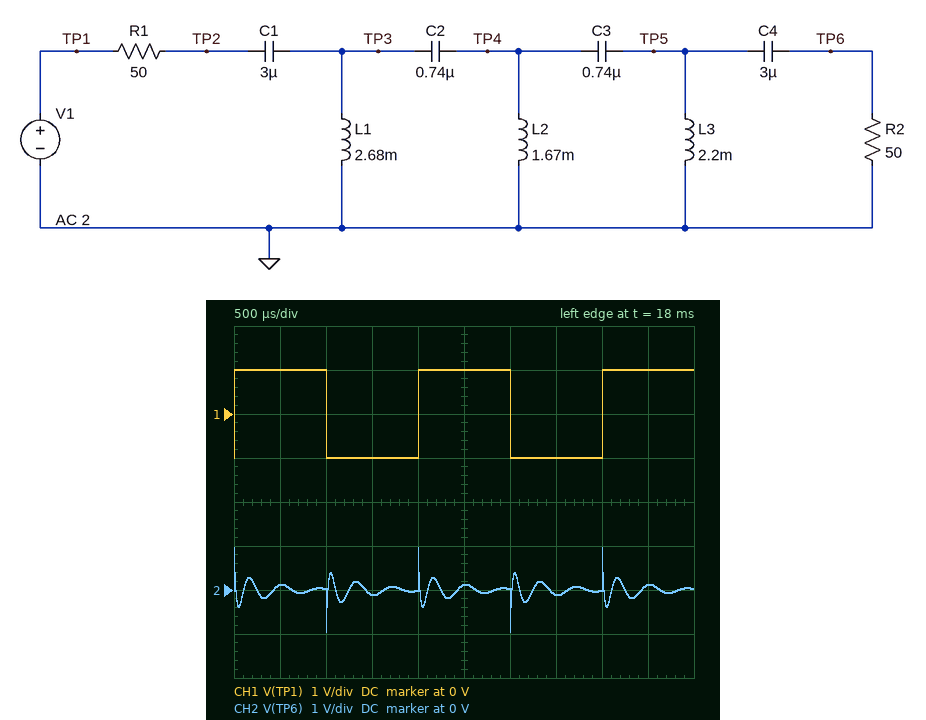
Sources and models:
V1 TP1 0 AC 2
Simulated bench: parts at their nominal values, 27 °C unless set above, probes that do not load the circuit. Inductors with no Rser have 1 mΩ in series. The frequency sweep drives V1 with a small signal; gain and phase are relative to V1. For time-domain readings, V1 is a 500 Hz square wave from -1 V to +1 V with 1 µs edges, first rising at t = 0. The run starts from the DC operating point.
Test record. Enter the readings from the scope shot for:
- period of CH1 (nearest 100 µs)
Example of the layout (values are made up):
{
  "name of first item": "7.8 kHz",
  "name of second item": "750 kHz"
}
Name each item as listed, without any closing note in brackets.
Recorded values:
{
  "period of CH1": "2.0 ms"
}
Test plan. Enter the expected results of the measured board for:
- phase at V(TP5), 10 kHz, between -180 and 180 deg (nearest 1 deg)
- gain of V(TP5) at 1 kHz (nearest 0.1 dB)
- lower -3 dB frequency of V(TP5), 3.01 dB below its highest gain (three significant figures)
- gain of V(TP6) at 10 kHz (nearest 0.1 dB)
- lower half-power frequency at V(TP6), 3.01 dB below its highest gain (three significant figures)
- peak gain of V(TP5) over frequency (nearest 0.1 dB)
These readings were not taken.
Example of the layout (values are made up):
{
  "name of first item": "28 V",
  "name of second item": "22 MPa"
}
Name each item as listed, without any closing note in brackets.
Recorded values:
{
  "phase at V(TP5), 10 kHz, between -180 and 180 deg": "58 deg",
  "gain of V(TP5) at 1 kHz": "-57.7 dB",
  "lower -3 dB frequency of V(TP5), 3.01 dB below its highest gain": "2.38 kHz",
  "gain of V(TP6) at 10 kHz": "-6.0 dB",
  "lower half-power frequency at V(TP6), 3.01 dB below its highest gain": "2.40 kHz",
  "peak gain of V(TP5) over frequency": "-5.5 dB"
}
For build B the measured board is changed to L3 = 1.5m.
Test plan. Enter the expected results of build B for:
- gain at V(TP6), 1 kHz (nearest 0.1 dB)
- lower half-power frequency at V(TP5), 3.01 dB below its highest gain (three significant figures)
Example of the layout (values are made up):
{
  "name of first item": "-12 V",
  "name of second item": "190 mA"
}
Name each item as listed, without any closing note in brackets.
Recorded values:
{
  "gain at V(TP6), 1 kHz": "-64.9 dB",
  "lower half-power frequency at V(TP5), 3.01 dB below its highest gain": "2.50 kHz"
}
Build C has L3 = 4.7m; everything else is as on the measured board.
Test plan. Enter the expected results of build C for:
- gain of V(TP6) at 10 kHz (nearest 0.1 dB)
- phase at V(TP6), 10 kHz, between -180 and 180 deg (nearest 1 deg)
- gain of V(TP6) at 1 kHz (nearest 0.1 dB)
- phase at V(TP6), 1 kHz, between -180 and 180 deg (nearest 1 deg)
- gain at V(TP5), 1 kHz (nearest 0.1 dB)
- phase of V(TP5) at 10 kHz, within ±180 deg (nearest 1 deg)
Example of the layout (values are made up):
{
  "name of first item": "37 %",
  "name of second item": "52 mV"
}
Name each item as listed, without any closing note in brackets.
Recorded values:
{
  "gain of V(TP6) at 10 kHz": "-6.0 dB",
  "phase at V(TP6), 10 kHz, between -180 and 180 deg": "58 deg",
  "gain of V(TP6) at 1 kHz": "-52.2 dB",
  "phase at V(TP6), 1 kHz, between -180 and 180 deg": "145 deg",
  "gain at V(TP5), 1 kHz": "-48.9 dB",
  "phase of V(TP5) at 10 kHz, within ±180 deg": "52 deg"
}
